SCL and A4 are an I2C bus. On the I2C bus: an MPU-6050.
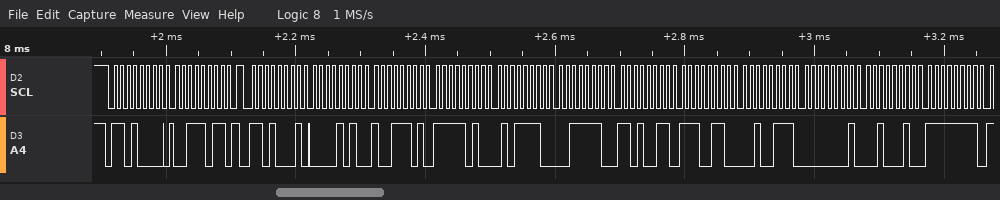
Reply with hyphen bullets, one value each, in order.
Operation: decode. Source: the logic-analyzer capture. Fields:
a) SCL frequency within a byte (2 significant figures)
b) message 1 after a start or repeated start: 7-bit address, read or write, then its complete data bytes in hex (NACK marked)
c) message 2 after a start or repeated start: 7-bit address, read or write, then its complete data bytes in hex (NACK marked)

- 100 kHz
- 0x68 write: 3B
- 0x68 read: 0A 9D FA 5E 3E D3 E6 27 01 22 FF
